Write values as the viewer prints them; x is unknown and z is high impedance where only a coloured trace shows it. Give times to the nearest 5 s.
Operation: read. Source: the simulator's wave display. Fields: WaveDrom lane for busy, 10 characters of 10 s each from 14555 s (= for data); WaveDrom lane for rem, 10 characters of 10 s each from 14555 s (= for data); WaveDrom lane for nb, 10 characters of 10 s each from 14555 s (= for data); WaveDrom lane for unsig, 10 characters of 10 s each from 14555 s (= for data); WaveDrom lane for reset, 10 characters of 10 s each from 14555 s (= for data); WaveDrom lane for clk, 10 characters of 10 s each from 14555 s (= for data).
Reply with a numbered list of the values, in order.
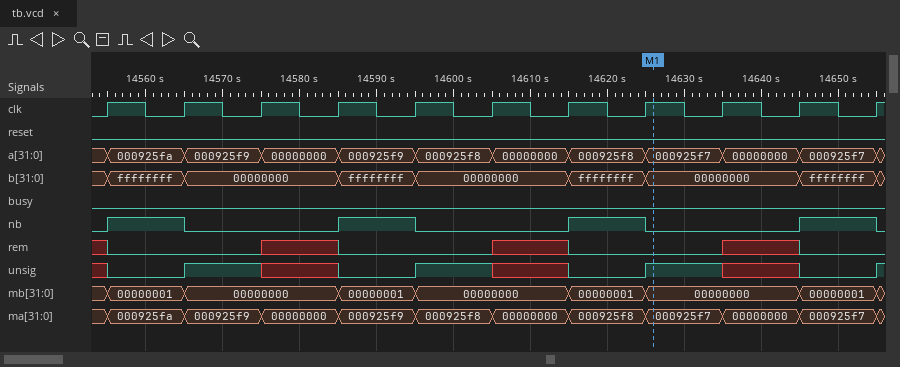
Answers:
1. {name: 'busy', wave: '0.........'}
2. {name: 'rem', wave: '0.x0.x0.x0'}
3. {name: 'nb', wave: '10.10.10.1'}
4. {name: 'unsig', wave: '01x01x01x0'}
5. {name: 'reset', wave: '0.........'}
6. {name: 'clk', wave: 'p.........'}
